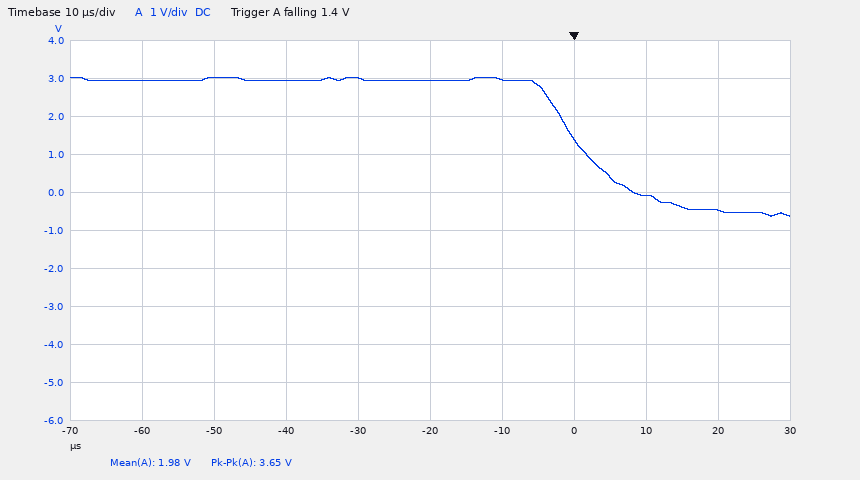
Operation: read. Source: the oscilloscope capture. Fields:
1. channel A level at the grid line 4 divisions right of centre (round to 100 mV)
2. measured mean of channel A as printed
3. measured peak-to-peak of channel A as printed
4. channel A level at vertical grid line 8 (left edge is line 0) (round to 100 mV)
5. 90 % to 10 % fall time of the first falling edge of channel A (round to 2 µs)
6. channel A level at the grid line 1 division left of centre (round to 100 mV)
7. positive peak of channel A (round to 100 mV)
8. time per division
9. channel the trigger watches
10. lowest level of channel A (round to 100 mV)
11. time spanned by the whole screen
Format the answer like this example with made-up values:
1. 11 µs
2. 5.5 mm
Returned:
1. -500 mV
2. 1.98 V
3. 3.65 V
4. -100 mV
5. 16 µs
6. 3.0 V
7. 3.0 V
8. 10 µs
9. channel A
10. -600 mV
11. 100 µs
